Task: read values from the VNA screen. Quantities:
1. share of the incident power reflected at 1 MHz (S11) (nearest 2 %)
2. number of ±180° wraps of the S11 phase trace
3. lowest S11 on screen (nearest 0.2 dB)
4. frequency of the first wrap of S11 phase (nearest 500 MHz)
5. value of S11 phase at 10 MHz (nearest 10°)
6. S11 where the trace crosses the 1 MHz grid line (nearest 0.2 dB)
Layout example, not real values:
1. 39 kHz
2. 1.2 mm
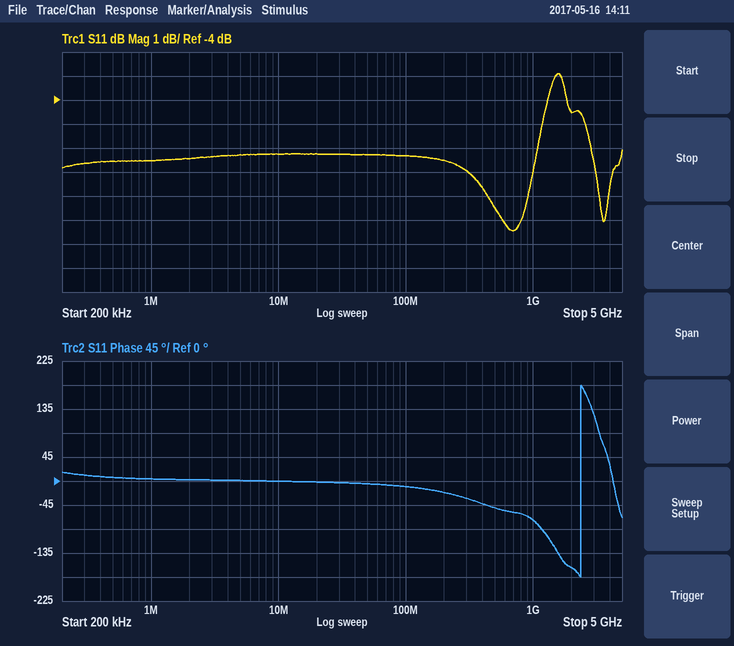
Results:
1. 22 %
2. 1
3. -9.4 dB
4. 2.5 GHz
5. 0°
6. -6.6 dB
